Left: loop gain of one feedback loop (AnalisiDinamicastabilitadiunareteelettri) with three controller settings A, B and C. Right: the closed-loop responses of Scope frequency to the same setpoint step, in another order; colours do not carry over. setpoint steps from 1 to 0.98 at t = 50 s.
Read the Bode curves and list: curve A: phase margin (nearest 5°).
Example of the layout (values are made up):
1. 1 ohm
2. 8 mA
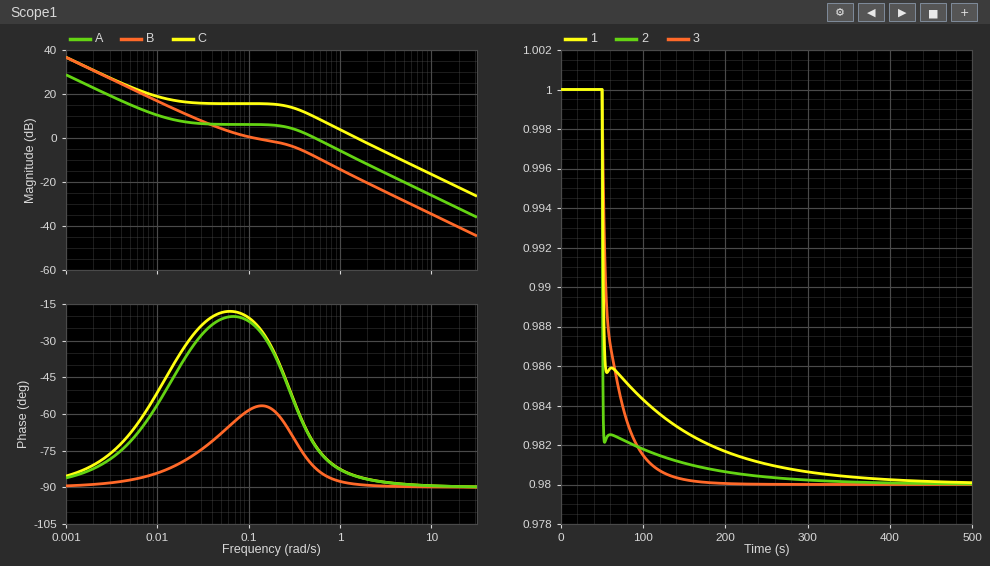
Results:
1. 105°
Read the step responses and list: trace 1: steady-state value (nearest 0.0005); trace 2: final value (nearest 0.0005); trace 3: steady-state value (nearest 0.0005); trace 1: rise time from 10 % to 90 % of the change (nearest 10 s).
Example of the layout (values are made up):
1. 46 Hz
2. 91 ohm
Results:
1. 0.9800
2. 0.9800
3. 0.9800
4. 130 s
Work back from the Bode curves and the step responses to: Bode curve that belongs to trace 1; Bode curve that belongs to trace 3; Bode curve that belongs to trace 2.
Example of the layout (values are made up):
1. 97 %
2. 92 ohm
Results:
1. A
2. B
3. C
